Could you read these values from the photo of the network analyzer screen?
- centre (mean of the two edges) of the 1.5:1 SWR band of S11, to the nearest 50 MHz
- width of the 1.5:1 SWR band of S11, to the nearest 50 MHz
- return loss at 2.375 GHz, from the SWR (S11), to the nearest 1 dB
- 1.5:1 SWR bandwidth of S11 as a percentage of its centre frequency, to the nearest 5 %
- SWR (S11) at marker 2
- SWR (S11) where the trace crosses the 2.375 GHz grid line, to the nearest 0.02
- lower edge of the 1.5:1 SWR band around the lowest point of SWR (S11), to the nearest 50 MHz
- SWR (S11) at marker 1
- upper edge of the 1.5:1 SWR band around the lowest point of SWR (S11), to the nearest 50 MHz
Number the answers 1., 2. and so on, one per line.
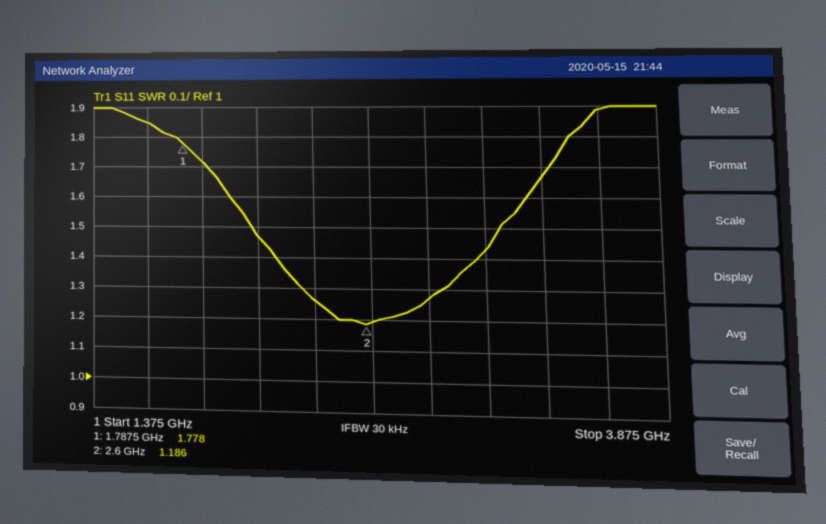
1. 2.65 GHz
2. 1.10 GHz
3. 19 dB
4. 40 %
5. 1.186
6. 1.26
7. 2.10 GHz
8. 1.778
9. 3.20 GHz
